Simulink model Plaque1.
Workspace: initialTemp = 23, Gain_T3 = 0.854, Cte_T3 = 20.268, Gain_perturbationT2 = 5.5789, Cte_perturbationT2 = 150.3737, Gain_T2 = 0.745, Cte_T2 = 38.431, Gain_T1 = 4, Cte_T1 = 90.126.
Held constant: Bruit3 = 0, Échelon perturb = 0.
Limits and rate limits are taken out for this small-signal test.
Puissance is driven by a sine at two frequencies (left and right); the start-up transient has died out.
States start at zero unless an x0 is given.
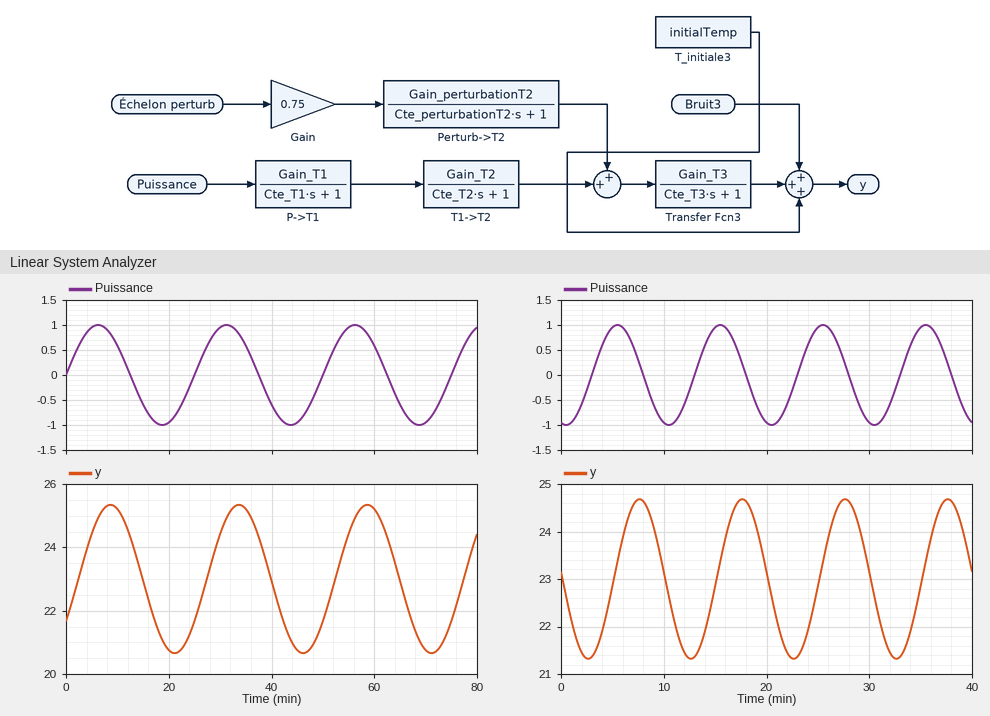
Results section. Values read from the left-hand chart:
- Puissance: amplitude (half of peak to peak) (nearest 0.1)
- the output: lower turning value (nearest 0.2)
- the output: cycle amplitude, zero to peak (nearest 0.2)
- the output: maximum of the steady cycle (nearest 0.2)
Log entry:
1.0
20.6
2.4
25.4
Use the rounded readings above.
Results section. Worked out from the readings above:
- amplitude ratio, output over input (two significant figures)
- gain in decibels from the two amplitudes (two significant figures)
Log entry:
2.4
7.6 dB
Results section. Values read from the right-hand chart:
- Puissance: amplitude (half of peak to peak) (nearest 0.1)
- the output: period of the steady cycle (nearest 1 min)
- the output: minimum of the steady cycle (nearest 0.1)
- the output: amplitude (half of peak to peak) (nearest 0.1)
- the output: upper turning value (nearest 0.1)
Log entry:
1.0
10 min
21.3
1.7
24.7
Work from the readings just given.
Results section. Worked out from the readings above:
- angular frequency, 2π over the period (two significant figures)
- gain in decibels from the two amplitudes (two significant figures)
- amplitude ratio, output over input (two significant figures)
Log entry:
0.63 rad/min
4.6 dB
1.7
